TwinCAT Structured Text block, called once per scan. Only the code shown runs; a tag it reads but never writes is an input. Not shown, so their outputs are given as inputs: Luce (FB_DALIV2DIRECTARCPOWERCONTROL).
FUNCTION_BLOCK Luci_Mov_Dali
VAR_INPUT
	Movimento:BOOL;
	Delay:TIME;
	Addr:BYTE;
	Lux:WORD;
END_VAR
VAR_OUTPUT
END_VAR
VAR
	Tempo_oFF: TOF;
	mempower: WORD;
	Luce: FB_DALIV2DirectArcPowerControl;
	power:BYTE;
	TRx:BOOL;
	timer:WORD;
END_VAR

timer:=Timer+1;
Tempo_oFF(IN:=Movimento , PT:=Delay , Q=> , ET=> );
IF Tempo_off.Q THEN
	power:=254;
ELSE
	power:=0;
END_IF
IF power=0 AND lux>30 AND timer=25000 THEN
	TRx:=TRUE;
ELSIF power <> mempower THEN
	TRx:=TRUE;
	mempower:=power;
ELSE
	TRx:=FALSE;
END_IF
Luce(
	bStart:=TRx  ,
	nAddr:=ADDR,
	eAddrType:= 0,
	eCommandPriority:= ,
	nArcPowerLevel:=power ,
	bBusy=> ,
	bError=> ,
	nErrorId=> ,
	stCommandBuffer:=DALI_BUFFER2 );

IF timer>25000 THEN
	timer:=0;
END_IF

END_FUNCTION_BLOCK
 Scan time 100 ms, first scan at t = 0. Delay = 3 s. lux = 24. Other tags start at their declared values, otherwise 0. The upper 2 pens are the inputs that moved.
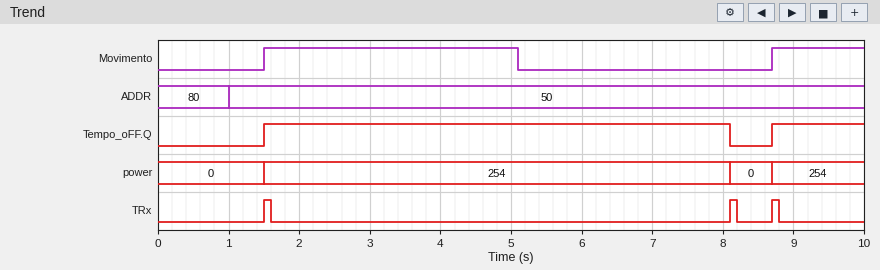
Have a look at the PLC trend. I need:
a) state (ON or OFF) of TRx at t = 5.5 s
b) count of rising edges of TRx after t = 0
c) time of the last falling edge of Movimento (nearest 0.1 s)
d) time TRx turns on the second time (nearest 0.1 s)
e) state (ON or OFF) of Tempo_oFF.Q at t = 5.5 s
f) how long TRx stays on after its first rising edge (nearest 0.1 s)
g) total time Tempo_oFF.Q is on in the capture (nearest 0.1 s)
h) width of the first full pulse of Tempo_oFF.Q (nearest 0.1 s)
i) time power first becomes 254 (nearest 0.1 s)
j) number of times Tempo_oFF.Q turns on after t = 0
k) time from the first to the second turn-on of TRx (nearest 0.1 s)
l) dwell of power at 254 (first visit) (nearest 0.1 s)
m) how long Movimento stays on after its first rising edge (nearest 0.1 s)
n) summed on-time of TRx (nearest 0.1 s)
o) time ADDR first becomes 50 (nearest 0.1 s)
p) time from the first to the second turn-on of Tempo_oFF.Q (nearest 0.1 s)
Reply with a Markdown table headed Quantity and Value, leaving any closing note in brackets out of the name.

| Quantity | Value |
|---|---|
| state (ON or OFF) of TRx at t = 5.5 s | OFF |
| count of rising edges of TRx after t = 0 | 3 |
| time of the last falling edge of Movimento | 5.1 s |
| time TRx turns on the second time | 8.1 s |
| state (ON or OFF) of Tempo_oFF.Q at t = 5.5 s | ON |
| how long TRx stays on after its first rising edge | 0.1 s |
| total time Tempo_oFF.Q is on in the capture | 7.9 s |
| width of the first full pulse of Tempo_oFF.Q | 6.6 s |
| time power first becomes 254 | 1.5 s |
| number of times Tempo_oFF.Q turns on after t = 0 | 2 |
| time from the first to the second turn-on of TRx | 6.6 s |
| dwell of power at 254 (first visit) | 6.6 s |
| how long Movimento stays on after its first rising edge | 3.6 s |
| summed on-time of TRx | 0.3 s |
| time ADDR first becomes 50 | 1.0 s |
| time from the first to the second turn-on of Tempo_oFF.Q | 7.2 s |
